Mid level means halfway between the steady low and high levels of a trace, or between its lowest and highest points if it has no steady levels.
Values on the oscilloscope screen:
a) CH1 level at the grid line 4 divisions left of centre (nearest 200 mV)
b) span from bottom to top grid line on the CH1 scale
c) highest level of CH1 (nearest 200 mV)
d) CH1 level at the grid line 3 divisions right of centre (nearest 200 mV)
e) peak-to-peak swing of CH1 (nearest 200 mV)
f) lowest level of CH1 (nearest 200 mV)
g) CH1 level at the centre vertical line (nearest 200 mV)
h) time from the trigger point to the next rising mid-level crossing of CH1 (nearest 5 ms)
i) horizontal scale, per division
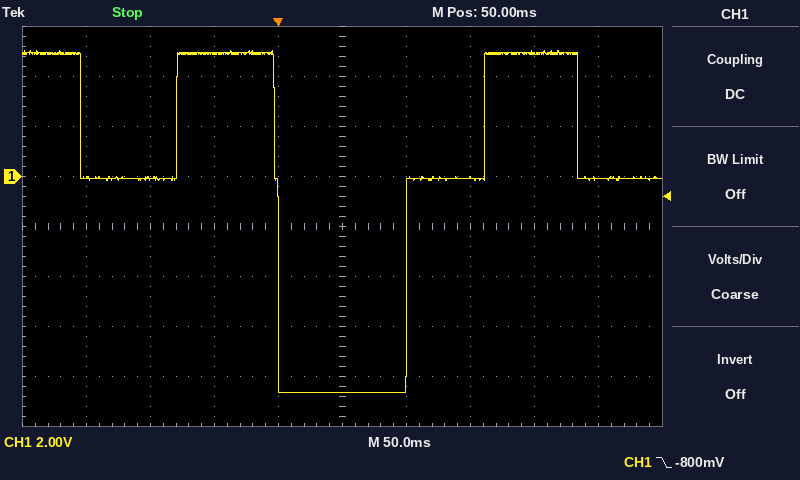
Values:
0.0 V
16 V
5.0 V
5.0 V
13.6 V
-8.6 V
-8.6 V
100 ms
50 ms
